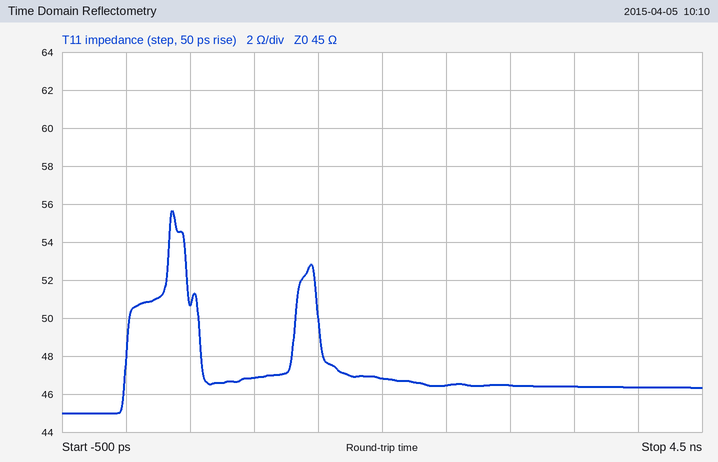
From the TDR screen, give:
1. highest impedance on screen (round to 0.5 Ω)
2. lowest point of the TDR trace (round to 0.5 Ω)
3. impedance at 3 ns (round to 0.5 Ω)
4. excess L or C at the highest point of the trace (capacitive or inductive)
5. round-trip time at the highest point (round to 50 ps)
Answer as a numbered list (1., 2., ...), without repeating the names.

1. 55.5 Ω
2. 45.0 Ω
3. 46.5 Ω
4. inductive
5. 350 ps
